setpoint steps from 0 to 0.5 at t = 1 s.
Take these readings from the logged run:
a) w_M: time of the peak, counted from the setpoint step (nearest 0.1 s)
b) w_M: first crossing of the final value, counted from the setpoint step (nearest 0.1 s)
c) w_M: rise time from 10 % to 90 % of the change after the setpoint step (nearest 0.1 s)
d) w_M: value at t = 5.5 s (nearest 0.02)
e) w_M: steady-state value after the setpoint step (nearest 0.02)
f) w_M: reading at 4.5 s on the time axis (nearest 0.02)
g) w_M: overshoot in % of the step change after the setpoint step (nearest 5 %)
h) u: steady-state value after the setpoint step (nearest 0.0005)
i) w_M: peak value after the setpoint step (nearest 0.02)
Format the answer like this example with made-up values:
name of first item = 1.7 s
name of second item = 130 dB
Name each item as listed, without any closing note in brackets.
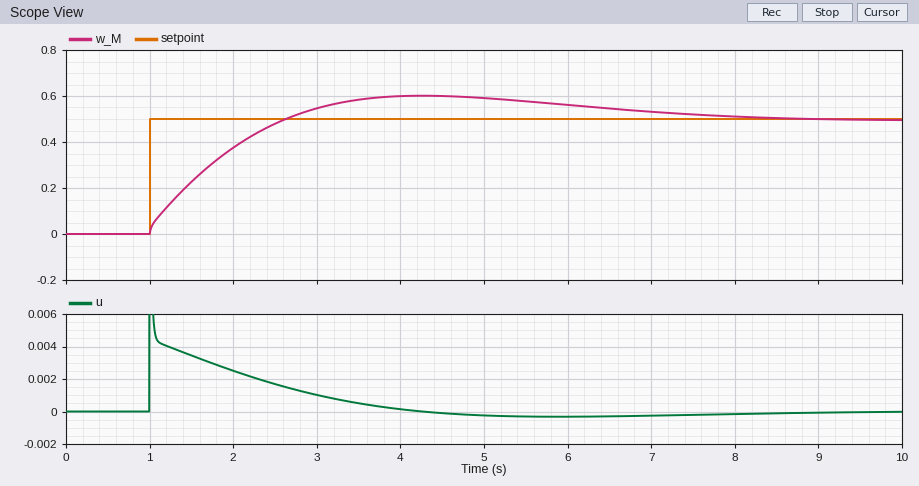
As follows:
w_M: time of the peak, counted from the setpoint step = 3.3 s
w_M: first crossing of the final value, counted from the setpoint step = 1.6 s
w_M: rise time from 10 % to 90 % of the change after the setpoint step = 1.3 s
w_M: value at t = 5.5 s = 0.58
w_M: steady-state value after the setpoint step = 0.50
w_M: reading at 4.5 s on the time axis = 0.60
w_M: overshoot in % of the step change after the setpoint step = 20 %
u: steady-state value after the setpoint step = 0.0000
w_M: peak value after the setpoint step = 0.60
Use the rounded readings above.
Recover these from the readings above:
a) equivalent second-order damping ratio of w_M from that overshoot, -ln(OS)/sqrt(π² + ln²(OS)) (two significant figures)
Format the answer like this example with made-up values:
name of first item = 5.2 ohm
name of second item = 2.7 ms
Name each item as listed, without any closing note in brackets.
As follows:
equivalent second-order damping ratio of w_M from that overshoot, -ln(OS)/sqrt(π² + ln²(OS)) = 0.46
